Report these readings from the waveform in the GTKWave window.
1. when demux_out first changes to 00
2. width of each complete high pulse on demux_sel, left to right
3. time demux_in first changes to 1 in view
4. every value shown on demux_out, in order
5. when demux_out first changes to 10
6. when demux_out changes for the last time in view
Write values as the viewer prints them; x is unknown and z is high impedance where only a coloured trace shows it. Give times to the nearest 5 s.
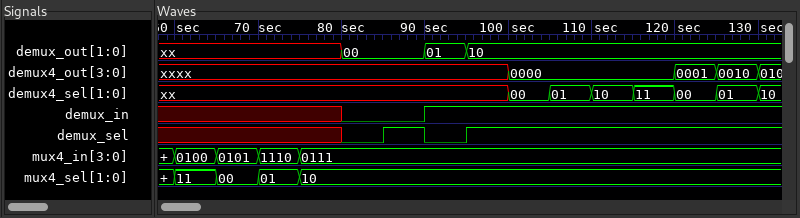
80 s
5 s
90 s
xx, 00, 01, 10
95 s
95 s
